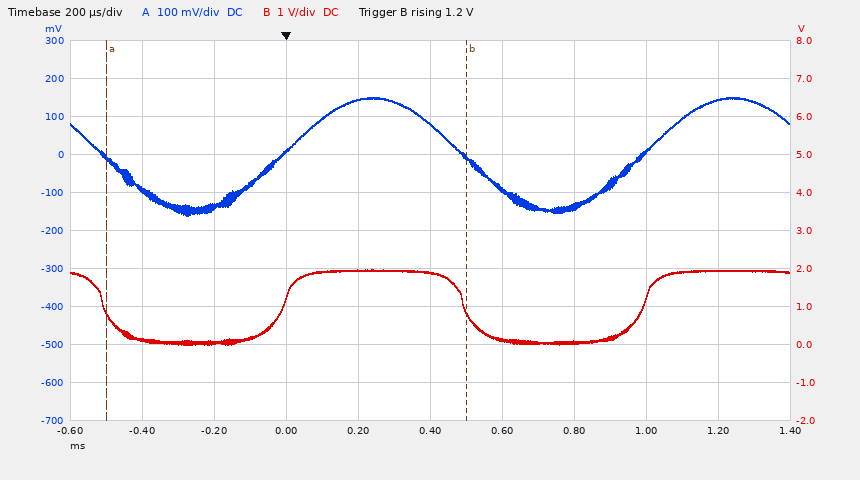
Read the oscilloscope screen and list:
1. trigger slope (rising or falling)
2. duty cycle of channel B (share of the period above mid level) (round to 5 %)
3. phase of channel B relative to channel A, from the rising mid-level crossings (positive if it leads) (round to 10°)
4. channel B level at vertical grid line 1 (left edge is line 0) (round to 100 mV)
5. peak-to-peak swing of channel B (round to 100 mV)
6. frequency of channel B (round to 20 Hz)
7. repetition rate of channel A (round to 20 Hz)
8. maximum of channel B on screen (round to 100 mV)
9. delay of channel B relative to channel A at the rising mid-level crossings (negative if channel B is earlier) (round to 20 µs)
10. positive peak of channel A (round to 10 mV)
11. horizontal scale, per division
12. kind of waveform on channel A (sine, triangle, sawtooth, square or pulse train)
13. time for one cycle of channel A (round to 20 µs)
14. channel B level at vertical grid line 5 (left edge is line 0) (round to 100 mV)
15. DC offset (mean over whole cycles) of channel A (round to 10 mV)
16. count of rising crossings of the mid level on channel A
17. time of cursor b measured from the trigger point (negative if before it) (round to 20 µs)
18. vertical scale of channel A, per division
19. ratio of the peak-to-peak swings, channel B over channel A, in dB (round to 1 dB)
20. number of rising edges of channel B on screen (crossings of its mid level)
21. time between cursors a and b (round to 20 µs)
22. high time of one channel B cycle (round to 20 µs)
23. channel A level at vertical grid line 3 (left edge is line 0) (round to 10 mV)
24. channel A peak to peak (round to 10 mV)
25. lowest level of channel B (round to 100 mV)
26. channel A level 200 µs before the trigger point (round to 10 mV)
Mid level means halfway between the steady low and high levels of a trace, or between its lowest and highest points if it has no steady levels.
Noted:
rising
50 %
0°
100 mV
2.0 V
1.00 kHz
1.00 kHz
2.0 V
0 µs
150 mV
200 µs
sine
1.00 ms
1.9 V
0 mV
2
+500 µs
100 mV
16 dB
2
1.00 ms
500 µs
10 mV
310 mV
0.0 V
-140 mV
